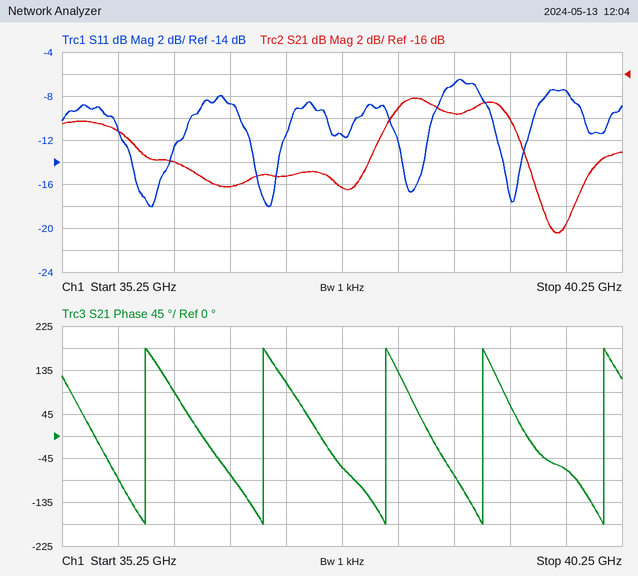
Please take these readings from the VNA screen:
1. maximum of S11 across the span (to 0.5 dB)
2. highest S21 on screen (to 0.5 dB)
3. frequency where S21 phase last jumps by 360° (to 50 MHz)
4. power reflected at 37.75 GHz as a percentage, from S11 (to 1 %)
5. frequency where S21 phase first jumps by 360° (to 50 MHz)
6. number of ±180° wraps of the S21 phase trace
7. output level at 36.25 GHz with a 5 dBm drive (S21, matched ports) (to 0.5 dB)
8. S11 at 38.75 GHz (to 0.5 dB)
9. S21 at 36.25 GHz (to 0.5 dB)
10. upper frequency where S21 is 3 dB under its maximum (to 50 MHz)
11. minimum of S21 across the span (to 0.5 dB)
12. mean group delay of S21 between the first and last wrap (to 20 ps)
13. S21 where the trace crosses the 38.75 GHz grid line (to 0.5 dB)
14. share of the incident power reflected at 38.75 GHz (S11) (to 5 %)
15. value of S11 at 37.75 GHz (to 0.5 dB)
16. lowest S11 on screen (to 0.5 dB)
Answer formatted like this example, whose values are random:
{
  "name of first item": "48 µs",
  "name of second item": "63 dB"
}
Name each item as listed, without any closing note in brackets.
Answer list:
{
  "maximum of S11 across the span": "-6.5 dB",
  "highest S21 on screen": "-18.0 dB",
  "frequency where S21 phase last jumps by 360°": "40.10 GHz",
  "power reflected at 37.75 GHz as a percentage, from S11": "7 %",
  "frequency where S21 phase first jumps by 360°": "36.00 GHz",
  "number of ±180° wraps of the S21 phase trace": "5",
  "output level at 36.25 GHz with a 5 dBm drive (S21, matched ports)": "-19.0 dBm",
  "S11 at 38.75 GHz": "-7.0 dB",
  "S21 at 36.25 GHz": "-24.0 dB",
  "upper frequency where S21 is 3 dB under its maximum": "39.30 GHz",
  "minimum of S21 across the span": "-30.5 dB",
  "mean group delay of S21 between the first and last wrap": "980 ps",
  "S21 where the trace crosses the 38.75 GHz grid line": "-19.5 dB",
  "share of the incident power reflected at 38.75 GHz (S11)": "20 %",
  "value of S11 at 37.75 GHz": "-11.5 dB",
  "lowest S11 on screen": "-18.0 dB"
}
